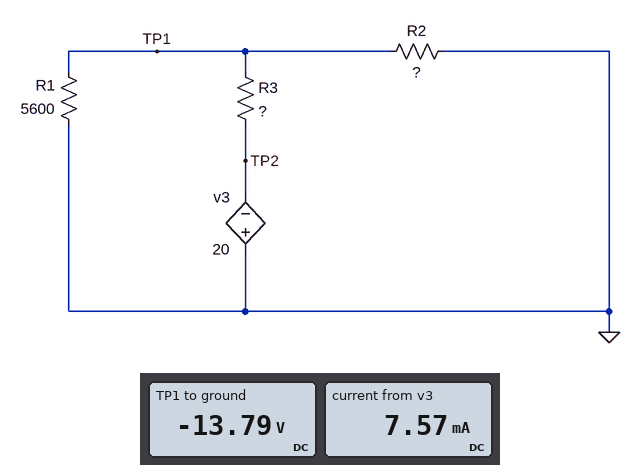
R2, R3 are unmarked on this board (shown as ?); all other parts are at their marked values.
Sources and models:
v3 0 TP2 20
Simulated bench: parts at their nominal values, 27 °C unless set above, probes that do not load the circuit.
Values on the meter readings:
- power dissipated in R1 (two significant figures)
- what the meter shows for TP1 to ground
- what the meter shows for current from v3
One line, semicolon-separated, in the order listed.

34 mW; -13.79 V; 7.57 mA
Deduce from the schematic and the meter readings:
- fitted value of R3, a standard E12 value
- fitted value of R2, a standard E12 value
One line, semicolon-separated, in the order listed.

820 Ω; 2.7 kΩ
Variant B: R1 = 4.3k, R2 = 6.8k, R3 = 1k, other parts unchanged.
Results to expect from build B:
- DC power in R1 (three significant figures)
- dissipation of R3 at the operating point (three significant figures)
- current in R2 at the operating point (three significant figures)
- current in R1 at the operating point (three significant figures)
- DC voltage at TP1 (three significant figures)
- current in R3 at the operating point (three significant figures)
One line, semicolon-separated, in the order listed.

48.9 mW; 30.3 mW; 2.13 mA; 3.37 mA; -14.5 V; 5.50 mA
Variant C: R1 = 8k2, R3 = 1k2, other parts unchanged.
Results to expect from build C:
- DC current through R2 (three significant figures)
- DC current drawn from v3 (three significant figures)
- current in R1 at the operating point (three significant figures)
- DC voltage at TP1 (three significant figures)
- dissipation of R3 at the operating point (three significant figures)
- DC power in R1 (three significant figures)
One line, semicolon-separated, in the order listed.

4.66 mA; 6.19 mA; 1.53 mA; -12.6 V; 46.0 mW; 19.3 mW
